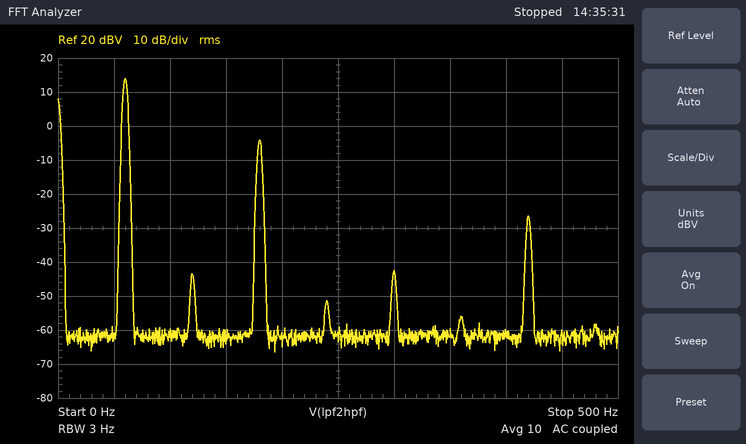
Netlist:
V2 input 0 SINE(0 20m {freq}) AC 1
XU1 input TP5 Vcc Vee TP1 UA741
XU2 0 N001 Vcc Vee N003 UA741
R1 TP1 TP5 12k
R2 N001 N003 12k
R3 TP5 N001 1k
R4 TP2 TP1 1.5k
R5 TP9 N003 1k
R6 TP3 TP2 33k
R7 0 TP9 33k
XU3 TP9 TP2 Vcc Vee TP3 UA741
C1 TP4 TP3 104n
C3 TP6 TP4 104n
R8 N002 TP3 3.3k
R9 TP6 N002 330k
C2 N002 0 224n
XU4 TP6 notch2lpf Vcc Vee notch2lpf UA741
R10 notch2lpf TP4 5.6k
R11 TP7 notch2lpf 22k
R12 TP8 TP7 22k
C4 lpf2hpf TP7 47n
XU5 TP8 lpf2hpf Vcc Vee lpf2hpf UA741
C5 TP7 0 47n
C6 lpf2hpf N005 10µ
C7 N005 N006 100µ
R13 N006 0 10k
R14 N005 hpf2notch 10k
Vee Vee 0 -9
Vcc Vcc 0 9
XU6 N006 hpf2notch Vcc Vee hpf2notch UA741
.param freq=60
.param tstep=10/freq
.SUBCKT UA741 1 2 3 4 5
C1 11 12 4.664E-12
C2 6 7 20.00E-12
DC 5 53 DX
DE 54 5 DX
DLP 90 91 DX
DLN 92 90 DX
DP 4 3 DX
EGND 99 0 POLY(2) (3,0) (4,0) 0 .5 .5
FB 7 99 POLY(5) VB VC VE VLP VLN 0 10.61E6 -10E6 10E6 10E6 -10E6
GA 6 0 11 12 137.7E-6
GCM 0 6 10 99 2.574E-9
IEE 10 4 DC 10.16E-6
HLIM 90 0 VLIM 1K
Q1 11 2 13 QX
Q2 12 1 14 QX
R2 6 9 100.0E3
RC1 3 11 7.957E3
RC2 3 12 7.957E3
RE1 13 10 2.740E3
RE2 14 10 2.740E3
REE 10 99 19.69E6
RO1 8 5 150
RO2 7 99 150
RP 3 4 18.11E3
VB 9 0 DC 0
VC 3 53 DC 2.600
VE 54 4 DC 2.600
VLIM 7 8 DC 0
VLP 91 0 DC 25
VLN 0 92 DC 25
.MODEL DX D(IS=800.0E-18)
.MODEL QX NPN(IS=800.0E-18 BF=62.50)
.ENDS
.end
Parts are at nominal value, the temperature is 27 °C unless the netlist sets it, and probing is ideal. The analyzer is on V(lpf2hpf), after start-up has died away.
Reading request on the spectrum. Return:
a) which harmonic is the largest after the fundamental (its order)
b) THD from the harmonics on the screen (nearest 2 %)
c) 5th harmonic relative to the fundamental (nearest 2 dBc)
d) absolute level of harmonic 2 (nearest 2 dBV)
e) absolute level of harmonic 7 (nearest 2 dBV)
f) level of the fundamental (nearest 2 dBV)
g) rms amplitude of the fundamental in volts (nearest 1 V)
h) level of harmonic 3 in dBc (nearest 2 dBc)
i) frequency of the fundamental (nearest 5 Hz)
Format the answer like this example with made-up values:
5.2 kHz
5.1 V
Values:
3
12 %
-56 dBc
-44 dBV
-26 dBV
14 dBV
5 V
-18 dBc
60 Hz
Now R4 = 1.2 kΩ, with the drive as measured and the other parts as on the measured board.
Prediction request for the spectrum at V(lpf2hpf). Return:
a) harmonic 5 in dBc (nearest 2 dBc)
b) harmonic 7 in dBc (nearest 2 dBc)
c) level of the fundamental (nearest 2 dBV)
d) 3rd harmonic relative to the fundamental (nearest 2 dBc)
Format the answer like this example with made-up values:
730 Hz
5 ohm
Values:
-32 dBc
-50 dBc
14 dBV
-16 dBc
